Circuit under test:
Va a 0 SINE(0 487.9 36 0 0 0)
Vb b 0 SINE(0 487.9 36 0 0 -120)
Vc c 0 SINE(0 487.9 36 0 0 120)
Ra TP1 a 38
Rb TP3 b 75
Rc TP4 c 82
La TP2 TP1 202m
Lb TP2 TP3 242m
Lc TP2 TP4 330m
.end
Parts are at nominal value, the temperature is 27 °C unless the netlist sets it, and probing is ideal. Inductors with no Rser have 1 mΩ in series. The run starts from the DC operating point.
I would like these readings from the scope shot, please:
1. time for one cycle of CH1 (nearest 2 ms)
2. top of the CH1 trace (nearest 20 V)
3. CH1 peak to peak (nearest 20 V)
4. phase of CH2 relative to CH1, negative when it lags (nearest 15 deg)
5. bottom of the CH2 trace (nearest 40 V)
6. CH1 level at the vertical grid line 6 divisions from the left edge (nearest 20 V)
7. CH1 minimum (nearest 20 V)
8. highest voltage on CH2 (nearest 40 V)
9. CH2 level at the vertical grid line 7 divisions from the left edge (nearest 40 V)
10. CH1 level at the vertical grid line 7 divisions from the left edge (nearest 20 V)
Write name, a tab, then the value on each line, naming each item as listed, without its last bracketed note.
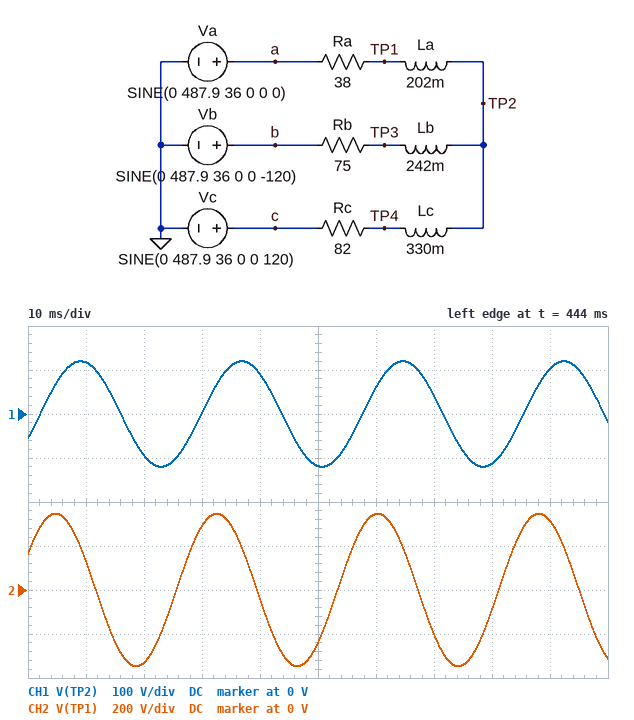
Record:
time for one cycle of CH1	28 ms
top of the CH1 trace	120 V
CH1 peak to peak	240 V
phase of CH2 relative to CH1, negative when it lags	60 deg
bottom of the CH2 trace	-360 V
CH1 level at the vertical grid line 6 divisions from the left edge	60 V
CH1 minimum	-120 V
highest voltage on CH2	360 V
CH2 level at the vertical grid line 7 divisions from the left edge	-200 V
CH1 level at the vertical grid line 7 divisions from the left edge	40 V
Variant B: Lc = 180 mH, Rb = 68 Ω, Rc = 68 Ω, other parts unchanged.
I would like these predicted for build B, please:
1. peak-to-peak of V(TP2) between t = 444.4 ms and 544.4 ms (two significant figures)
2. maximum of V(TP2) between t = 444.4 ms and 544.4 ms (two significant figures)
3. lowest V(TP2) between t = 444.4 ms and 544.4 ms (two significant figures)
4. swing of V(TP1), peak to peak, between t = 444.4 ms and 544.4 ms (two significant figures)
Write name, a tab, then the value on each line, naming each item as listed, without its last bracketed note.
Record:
peak-to-peak of V(TP2) between t = 444.4 ms and 544.4 ms	110 V
maximum of V(TP2) between t = 444.4 ms and 544.4 ms	54 V
lowest V(TP2) between t = 444.4 ms and 544.4 ms	-54 V
swing of V(TP1), peak to peak, between t = 444.4 ms and 544.4 ms	700 V
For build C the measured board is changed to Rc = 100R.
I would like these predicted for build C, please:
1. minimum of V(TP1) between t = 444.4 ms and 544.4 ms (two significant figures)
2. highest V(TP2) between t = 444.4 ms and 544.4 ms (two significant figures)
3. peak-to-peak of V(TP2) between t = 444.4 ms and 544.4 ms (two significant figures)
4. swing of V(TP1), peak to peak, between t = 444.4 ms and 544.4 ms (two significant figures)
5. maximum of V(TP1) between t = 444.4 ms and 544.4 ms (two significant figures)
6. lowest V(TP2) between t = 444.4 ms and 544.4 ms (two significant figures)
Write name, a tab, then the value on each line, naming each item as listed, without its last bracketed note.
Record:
minimum of V(TP1) between t = 444.4 ms and 544.4 ms	-330 V
highest V(TP2) between t = 444.4 ms and 544.4 ms	130 V
peak-to-peak of V(TP2) between t = 444.4 ms and 544.4 ms	260 V
swing of V(TP1), peak to peak, between t = 444.4 ms and 544.4 ms	670 V
maximum of V(TP1) between t = 444.4 ms and 544.4 ms	330 V
lowest V(TP2) between t = 444.4 ms and 544.4 ms	-130 V
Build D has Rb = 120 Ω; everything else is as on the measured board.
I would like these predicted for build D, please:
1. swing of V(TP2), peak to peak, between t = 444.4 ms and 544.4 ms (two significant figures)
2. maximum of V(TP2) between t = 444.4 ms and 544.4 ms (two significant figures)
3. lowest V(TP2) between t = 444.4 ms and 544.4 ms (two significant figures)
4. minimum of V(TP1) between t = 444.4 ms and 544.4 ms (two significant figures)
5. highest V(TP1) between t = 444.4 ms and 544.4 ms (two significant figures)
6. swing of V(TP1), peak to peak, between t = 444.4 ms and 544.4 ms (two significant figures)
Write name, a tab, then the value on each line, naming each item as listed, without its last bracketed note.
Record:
swing of V(TP2), peak to peak, between t = 444.4 ms and 544.4 ms	320 V
maximum of V(TP2) between t = 444.4 ms and 544.4 ms	160 V
lowest V(TP2) between t = 444.4 ms and 544.4 ms	-160 V
minimum of V(TP1) between t = 444.4 ms and 544.4 ms	-370 V
highest V(TP1) between t = 444.4 ms and 544.4 ms	370 V
swing of V(TP1), peak to peak, between t = 444.4 ms and 544.4 ms	740 V
